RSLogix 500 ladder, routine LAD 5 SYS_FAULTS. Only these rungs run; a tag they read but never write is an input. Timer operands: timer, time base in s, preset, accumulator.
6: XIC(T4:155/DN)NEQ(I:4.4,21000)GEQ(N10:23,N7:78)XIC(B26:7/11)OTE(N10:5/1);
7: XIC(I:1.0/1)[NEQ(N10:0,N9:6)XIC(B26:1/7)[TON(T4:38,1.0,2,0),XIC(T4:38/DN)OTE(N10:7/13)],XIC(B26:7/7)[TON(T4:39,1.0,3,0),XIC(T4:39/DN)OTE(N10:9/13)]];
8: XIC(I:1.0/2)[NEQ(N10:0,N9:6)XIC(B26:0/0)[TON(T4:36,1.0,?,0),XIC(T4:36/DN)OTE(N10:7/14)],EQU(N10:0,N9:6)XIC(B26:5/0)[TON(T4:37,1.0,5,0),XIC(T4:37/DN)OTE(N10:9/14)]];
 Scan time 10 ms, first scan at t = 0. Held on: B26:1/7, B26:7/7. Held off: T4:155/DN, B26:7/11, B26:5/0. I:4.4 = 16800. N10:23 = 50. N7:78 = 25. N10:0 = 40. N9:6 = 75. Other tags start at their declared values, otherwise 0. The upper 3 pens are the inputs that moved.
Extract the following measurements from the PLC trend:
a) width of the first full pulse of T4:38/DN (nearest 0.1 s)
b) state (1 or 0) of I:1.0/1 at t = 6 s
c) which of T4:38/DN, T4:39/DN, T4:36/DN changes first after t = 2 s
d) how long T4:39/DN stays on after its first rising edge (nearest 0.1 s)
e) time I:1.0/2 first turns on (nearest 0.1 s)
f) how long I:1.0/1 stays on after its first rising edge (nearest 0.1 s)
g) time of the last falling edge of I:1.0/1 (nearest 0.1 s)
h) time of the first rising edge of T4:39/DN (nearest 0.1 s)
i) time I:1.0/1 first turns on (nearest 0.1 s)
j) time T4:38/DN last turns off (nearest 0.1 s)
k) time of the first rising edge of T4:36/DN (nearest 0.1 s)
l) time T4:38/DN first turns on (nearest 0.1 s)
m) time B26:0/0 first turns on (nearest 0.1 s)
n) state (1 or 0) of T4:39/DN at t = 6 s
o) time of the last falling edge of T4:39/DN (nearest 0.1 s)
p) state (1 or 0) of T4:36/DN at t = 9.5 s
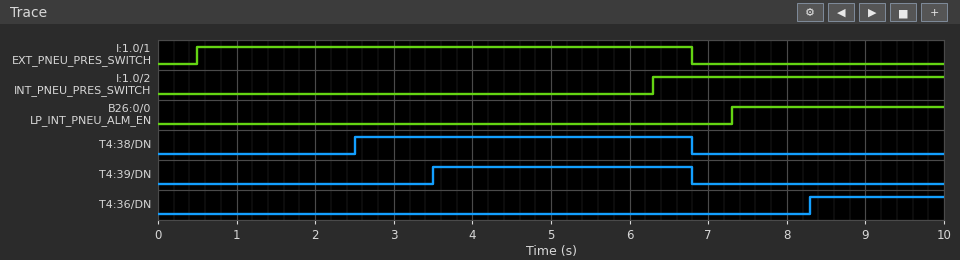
4.3 s
1
T4:38/DN
3.3 s
6.3 s
6.3 s
6.8 s
3.5 s
0.5 s
6.8 s
8.3 s
2.5 s
7.3 s
1
6.8 s
1
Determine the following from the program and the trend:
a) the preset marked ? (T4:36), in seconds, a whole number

1 s
